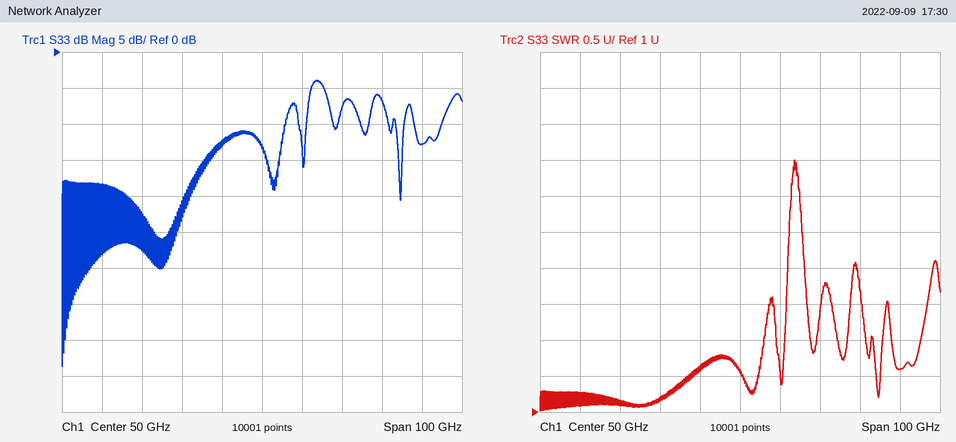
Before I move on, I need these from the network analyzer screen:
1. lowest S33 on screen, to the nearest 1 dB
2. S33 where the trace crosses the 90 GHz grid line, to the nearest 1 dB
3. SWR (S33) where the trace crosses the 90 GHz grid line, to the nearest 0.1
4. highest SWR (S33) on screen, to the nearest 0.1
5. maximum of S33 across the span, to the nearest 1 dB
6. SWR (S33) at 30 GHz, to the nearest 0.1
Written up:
-44 dB
-13 dB
1.6
4.5
-4 dB
1.2
